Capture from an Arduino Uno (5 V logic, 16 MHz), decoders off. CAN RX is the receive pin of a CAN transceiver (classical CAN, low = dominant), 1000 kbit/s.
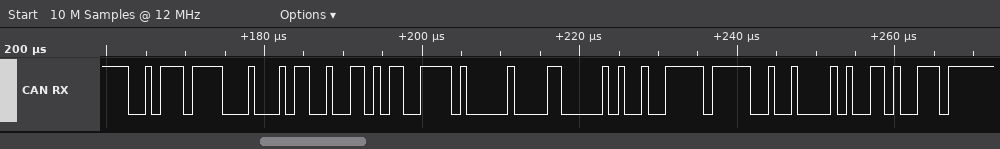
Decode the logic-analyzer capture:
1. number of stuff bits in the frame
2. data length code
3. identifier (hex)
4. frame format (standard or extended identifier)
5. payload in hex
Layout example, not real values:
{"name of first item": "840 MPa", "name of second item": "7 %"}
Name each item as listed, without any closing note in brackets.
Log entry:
{"number of stuff bits in the frame": "4", "data length code": "8", "identifier": "0x2EF", "frame format": "standard", "payload in hex": "B2 6B 3D 00 60 49 FF A4"}
